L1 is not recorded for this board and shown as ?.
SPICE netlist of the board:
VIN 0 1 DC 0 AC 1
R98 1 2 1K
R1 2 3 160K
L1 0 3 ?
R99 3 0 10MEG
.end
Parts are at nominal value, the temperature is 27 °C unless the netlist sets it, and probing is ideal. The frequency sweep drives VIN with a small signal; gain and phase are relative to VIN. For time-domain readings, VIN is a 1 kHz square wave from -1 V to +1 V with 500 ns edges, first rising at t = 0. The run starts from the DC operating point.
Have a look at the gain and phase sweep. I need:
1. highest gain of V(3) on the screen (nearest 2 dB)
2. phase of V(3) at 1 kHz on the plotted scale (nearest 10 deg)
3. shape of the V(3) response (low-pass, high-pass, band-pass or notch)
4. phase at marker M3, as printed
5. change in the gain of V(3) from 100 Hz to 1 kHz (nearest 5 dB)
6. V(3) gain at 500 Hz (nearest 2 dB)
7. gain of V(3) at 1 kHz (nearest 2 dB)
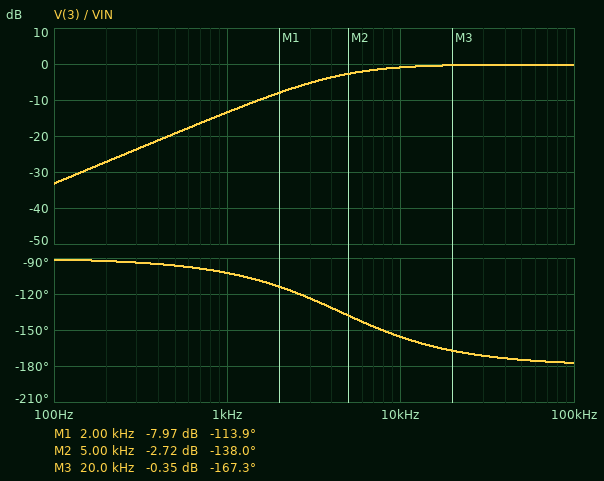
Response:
0 dB
-100 deg
high-pass
-167.3 deg
20 dB
-20 dB
-14 dB
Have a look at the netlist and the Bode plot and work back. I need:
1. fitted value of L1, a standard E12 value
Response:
5.6 H
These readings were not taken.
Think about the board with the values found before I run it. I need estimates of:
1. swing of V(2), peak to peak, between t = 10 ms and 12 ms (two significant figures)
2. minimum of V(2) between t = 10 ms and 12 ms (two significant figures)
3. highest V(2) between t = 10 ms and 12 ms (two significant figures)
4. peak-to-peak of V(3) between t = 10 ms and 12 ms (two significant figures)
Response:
2.0 V
-1.0 V
1.0 V
3.9 V
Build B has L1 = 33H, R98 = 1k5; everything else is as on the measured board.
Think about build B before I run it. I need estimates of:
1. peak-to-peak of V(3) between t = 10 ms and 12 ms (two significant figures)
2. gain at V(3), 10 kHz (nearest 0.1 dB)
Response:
3.6 V
-0.2 dB
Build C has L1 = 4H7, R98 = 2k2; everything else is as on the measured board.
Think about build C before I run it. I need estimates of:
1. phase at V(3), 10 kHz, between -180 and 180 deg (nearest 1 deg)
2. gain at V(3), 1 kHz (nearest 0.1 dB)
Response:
-152 deg
-14.9 dB
